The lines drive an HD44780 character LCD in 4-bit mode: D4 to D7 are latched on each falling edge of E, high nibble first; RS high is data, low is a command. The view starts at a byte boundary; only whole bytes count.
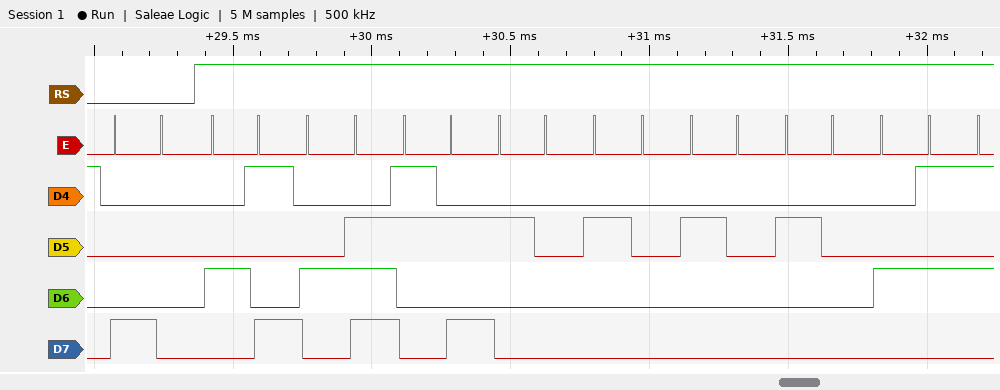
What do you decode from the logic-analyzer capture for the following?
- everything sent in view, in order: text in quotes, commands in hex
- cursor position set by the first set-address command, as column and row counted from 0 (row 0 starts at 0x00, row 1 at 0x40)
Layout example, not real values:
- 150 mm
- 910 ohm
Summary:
- 0x80 "IN:    E"
- column 0, row 0
